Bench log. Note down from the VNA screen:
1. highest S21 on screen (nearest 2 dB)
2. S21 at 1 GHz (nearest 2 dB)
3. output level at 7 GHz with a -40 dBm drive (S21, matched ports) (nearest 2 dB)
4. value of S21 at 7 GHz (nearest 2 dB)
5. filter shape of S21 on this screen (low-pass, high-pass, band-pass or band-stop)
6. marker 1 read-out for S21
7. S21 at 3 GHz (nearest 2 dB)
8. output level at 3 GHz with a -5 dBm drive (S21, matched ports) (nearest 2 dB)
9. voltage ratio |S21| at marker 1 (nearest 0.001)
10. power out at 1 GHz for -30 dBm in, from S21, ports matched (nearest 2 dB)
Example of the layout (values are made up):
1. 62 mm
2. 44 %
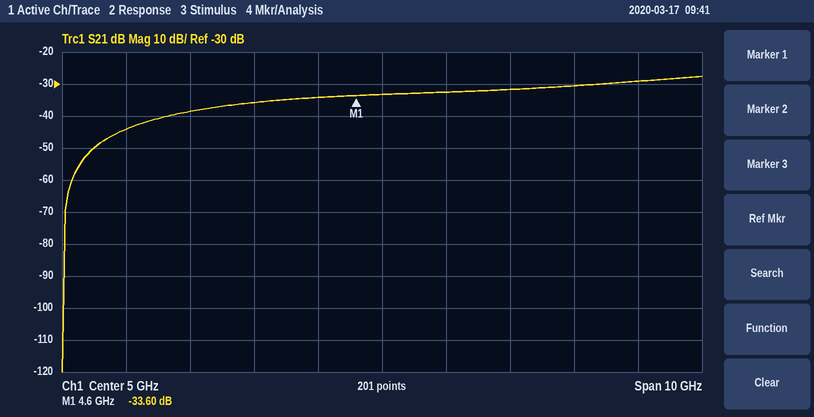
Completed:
1. -28 dB
2. -44 dB
3. -72 dBm
4. -32 dB
5. high-pass
6. -33.60 dB
7. -36 dB
8. -40 dBm
9. 0.021
10. -74 dBm
